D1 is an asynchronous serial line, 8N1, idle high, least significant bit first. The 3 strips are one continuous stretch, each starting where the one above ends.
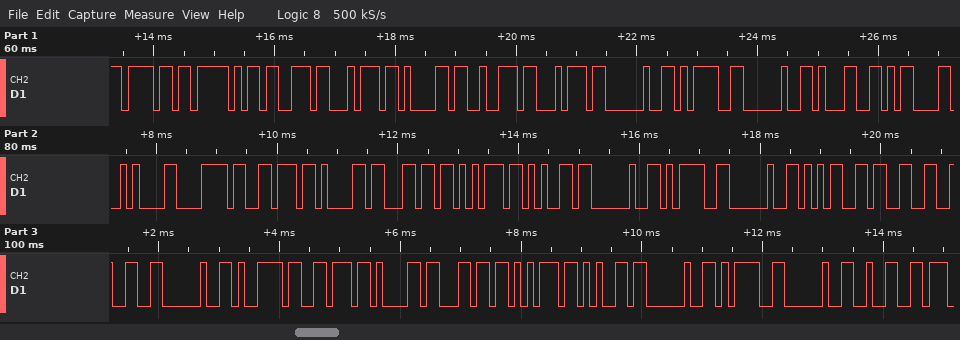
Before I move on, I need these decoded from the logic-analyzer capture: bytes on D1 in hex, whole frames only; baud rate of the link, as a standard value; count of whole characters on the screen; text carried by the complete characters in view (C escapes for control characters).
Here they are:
6F 5F 73 74 61 72 74 20 3D 20 31 0D 0A 78 76 61 6C 75 65 20 3D 20 35 33 32 20 79 76 61 6C 75 65 20 3D 20 32
9600 baud
36
"o_start = 1\r\nxvalue = 532 yvalue = 2"
